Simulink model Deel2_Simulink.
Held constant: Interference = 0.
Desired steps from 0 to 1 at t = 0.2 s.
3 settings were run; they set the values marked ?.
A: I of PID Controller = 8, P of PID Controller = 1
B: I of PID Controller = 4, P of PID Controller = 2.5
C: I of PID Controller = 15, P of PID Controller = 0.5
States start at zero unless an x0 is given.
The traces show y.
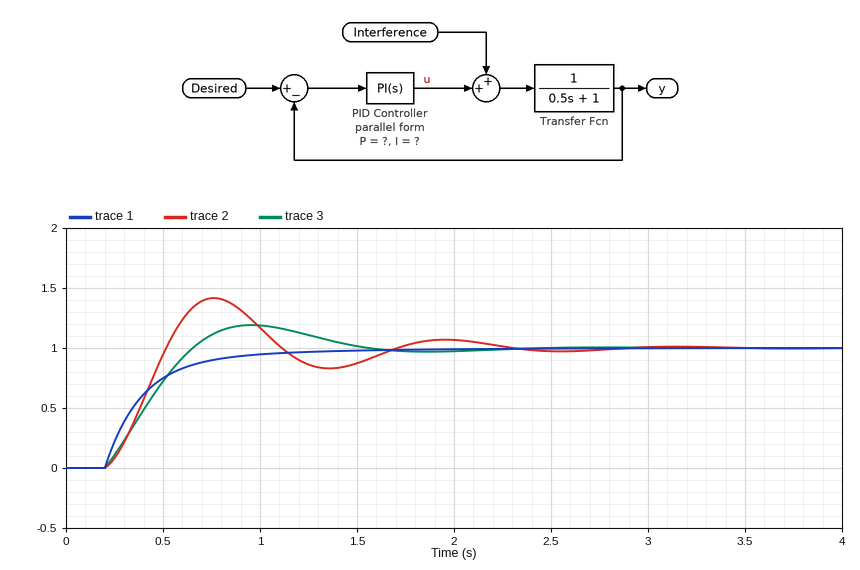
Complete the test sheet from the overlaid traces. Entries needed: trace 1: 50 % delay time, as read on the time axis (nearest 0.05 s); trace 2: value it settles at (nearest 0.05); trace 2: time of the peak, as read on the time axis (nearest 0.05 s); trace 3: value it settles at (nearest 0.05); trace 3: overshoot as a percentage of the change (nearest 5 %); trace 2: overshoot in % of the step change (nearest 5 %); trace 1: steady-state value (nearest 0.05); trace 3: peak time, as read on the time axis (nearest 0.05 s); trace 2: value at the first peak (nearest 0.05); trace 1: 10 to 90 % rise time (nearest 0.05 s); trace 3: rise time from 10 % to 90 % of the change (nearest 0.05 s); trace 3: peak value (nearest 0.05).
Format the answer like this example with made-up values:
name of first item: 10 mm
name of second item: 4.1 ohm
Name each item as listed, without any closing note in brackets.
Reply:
trace 1: 50 % delay time, as read on the time axis: 0.35 s
trace 2: value it settles at: 1.00
trace 2: time of the peak, as read on the time axis: 0.75 s
trace 3: value it settles at: 1.00
trace 3: overshoot as a percentage of the change: 20 %
trace 2: overshoot in % of the step change: 40 %
trace 1: steady-state value: 1.00
trace 3: peak time, as read on the time axis: 0.95 s
trace 2: value at the first peak: 1.40
trace 1: 10 to 90 % rise time: 0.55 s
trace 3: rise time from 10 % to 90 % of the change: 0.35 s
trace 3: peak value: 1.20
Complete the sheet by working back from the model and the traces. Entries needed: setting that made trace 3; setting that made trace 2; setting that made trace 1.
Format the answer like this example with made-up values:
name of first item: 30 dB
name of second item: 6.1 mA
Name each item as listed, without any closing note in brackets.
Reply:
setting that made trace 3: A
setting that made trace 2: C
setting that made trace 1: B
